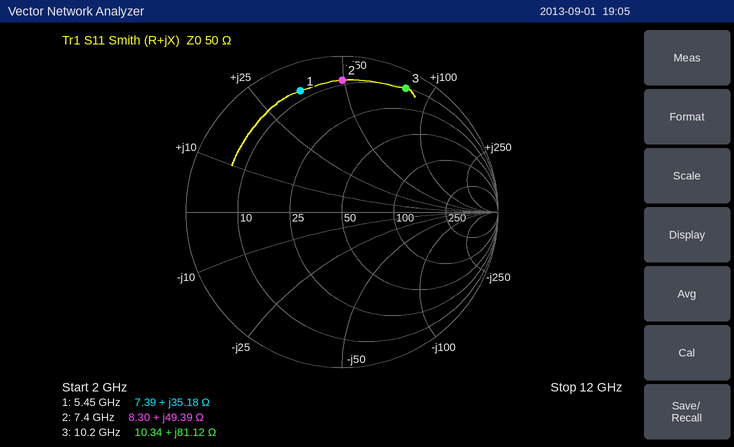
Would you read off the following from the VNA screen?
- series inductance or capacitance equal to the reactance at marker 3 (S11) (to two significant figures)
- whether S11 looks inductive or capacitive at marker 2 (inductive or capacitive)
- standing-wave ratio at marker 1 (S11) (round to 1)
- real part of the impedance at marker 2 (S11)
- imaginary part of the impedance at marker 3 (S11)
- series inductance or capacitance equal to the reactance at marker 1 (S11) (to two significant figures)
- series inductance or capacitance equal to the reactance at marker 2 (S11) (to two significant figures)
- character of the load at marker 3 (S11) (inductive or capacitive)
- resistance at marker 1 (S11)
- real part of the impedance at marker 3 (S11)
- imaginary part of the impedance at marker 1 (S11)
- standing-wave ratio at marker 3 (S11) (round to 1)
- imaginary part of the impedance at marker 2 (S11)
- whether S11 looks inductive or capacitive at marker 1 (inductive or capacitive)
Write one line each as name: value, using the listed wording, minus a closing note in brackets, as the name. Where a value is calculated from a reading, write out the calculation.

series inductance or capacitance equal to the reactance at marker 3 (S11): L = 81.12 Ω/(2π × 10.2 GHz) ≈ 1.3 nH
whether S11 looks inductive or capacitive at marker 2: inductive
standing-wave ratio at marker 1 (S11): 10
real part of the impedance at marker 2: 8.30 Ω
imaginary part of the impedance at marker 3: +81.12 Ω
series inductance or capacitance equal to the reactance at marker 1 (S11): L = 35.18 Ω/(2π × 5.45 GHz) ≈ 1.0 nH
series inductance or capacitance equal to the reactance at marker 2 (S11): L = 49.39 Ω/(2π × 7.4 GHz) ≈ 1.1 nH
character of the load at marker 3 (S11): inductive
resistance at marker 1: 7.39 Ω
real part of the impedance at marker 3: 10.34 Ω
imaginary part of the impedance at marker 1: +35.18 Ω
standing-wave ratio at marker 3 (S11): 18
imaginary part of the impedance at marker 2: +49.39 Ω
whether S11 looks inductive or capacitive at marker 1: inductive
